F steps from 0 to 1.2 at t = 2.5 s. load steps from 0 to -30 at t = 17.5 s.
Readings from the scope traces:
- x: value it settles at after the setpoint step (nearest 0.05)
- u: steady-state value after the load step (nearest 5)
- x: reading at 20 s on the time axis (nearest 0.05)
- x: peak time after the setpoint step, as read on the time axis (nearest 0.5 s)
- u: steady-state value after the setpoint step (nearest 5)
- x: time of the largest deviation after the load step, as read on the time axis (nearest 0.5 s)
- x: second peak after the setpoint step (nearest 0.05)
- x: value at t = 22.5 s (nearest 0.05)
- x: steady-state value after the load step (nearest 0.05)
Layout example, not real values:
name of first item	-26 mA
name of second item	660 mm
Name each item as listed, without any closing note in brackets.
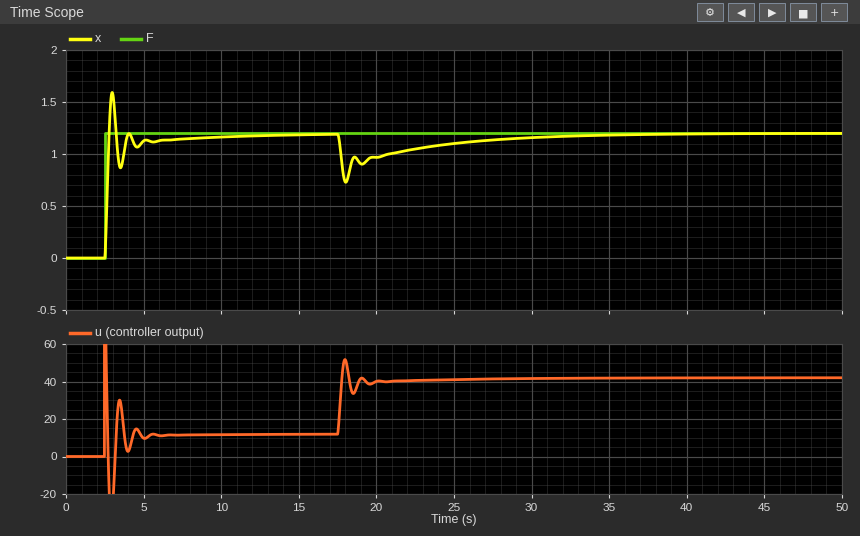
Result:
x: value it settles at after the setpoint step	1.20
u: steady-state value after the load step	40
x: reading at 20 s on the time axis	0.95
x: peak time after the setpoint step, as read on the time axis	3.0 s
u: steady-state value after the setpoint step	10
x: time of the largest deviation after the load step, as read on the time axis	18.0 s
x: second peak after the setpoint step	1.20
x: value at t = 22.5 s	1.05
x: steady-state value after the load step	1.20
